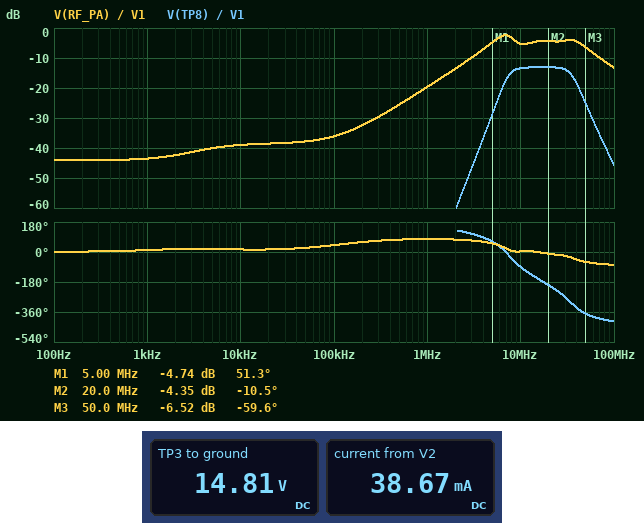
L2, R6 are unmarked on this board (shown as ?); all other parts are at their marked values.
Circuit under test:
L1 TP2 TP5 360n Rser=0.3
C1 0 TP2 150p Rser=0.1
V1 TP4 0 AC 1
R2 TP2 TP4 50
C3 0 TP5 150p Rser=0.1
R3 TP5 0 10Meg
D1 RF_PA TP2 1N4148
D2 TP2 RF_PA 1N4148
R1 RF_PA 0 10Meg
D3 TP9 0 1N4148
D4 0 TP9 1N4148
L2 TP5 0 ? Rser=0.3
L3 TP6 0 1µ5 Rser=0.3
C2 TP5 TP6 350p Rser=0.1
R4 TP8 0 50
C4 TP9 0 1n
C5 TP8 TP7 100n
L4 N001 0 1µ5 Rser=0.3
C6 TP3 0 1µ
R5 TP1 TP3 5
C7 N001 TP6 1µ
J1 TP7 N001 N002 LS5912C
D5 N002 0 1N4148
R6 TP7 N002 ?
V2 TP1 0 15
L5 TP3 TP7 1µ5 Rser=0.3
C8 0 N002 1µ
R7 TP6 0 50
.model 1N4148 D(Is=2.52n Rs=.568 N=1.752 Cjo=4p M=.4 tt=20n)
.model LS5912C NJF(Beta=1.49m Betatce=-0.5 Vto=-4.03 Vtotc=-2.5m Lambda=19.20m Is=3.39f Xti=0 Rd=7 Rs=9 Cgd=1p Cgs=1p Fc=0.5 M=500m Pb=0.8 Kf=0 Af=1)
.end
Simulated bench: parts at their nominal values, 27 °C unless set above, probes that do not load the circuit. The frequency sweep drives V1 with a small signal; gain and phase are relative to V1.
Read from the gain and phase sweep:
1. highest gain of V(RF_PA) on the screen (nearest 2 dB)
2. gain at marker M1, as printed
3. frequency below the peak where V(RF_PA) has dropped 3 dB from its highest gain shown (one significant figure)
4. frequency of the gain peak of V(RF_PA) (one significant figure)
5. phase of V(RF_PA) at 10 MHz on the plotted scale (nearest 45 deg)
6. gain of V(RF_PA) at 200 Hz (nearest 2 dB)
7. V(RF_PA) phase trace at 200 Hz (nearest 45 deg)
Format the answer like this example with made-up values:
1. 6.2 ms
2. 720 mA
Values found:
1. -2 dB
2. -4.74 dB
3. 5 MHz
4. 7 MHz
5. 0 deg
6. -44 dB
7. 0 deg
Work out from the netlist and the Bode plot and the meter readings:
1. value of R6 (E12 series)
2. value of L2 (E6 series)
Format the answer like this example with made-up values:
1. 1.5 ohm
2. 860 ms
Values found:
1. 680 Ω
2. 470 nH
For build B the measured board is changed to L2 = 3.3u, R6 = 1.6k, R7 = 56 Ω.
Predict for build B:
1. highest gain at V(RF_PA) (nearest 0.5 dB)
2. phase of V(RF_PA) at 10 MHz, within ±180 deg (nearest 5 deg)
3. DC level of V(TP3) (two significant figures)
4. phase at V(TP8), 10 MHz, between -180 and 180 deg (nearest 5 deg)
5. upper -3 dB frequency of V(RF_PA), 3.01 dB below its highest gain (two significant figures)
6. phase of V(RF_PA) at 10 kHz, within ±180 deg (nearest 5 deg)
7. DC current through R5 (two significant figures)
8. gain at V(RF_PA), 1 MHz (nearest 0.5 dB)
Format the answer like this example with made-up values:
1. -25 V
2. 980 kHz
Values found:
1. 0 dB
2. 0 deg
3. 15 V
4. -120 deg
5. 5.3 MHz
6. 30 deg
7. 27 mA
8. -7.0 dB
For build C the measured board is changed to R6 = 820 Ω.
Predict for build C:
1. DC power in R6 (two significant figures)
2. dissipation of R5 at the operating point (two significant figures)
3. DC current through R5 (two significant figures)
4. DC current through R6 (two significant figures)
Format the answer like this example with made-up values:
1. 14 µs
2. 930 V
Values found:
1. 240 mW
2. 6.2 mW
3. 35 mA
4. 17 mA
